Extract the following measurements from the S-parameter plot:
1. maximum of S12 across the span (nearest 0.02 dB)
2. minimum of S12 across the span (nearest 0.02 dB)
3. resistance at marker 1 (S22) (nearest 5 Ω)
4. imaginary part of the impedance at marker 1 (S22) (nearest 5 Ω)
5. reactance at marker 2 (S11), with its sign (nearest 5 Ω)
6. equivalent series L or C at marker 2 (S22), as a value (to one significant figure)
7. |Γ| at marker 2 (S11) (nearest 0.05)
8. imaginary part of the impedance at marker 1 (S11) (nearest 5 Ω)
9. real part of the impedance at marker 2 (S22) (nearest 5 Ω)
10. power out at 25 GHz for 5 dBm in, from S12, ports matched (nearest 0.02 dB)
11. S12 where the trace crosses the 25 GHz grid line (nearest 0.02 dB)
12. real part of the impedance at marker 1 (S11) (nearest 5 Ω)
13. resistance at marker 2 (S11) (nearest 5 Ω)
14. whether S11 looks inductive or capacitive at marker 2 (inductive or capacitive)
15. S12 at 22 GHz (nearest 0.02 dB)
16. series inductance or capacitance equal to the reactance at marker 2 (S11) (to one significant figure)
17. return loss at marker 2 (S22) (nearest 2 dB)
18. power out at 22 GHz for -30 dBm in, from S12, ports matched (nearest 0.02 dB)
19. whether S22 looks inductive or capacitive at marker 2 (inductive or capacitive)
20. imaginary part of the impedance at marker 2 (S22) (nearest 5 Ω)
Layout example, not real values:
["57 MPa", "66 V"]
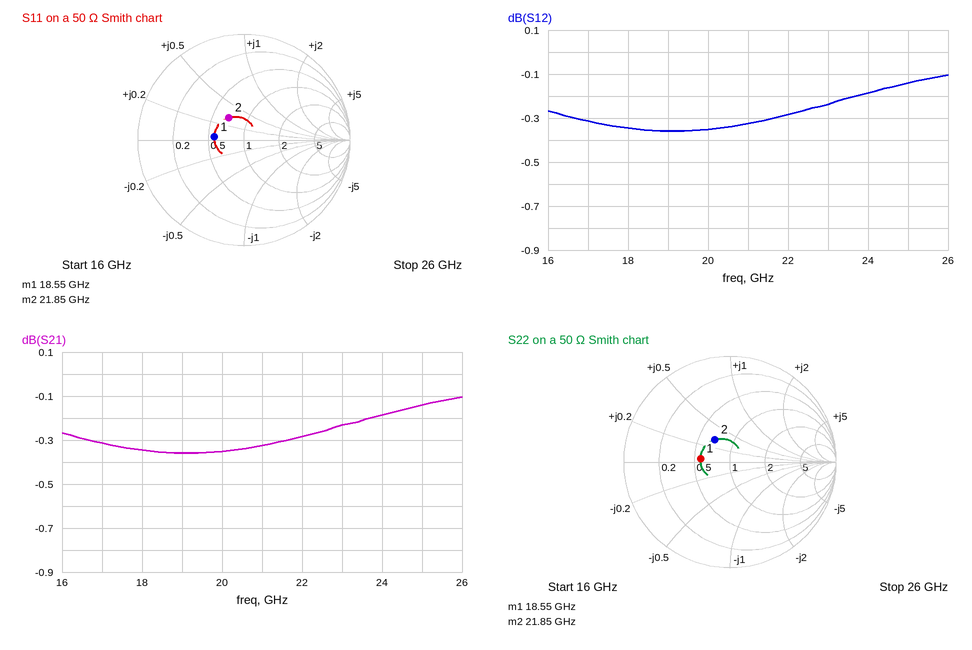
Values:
["-0.10 dB", "-0.36 dB", "30 Ω", "0 Ω", "+15 Ω", "100 pH", "0.25", "0 Ω", "35 Ω", "4.86 dBm", "-0.14 dB", "30 Ω", "35 Ω", "inductive", "-0.28 dB", "100 pH", "12 dB", "-30.28 dBm", "inductive", "+15 Ω"]
